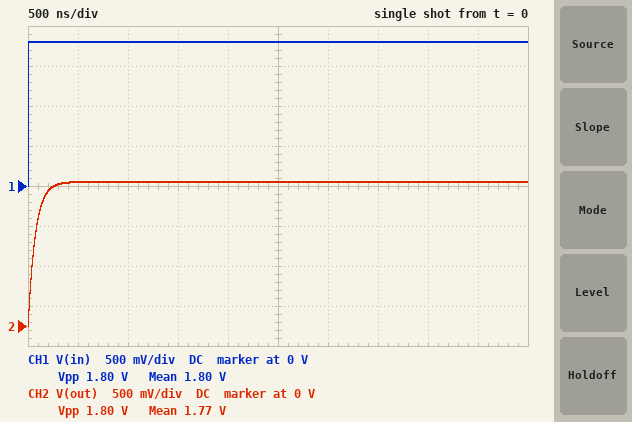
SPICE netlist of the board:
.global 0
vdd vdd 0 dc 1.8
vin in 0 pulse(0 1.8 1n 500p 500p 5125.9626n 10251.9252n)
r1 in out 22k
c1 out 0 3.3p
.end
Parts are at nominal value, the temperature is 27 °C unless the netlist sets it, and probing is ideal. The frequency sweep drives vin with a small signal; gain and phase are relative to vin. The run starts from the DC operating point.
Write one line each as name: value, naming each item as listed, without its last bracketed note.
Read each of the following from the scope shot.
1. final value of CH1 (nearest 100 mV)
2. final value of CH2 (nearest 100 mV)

final value of CH1: 1.8 V
final value of CH2: 1.8 V
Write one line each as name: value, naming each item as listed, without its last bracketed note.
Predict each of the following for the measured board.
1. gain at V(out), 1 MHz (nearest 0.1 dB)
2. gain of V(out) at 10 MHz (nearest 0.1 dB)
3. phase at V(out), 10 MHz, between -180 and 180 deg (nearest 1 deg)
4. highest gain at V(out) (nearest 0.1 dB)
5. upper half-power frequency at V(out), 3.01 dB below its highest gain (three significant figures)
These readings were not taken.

gain at V(out), 1 MHz: -0.8 dB
gain of V(out) at 10 MHz: -13.4 dB
phase at V(out), 10 MHz, between -180 and 180 deg: -78 deg
highest gain at V(out): 0 dB
upper half-power frequency at V(out), 3.01 dB below its highest gain: 2.19 MHz
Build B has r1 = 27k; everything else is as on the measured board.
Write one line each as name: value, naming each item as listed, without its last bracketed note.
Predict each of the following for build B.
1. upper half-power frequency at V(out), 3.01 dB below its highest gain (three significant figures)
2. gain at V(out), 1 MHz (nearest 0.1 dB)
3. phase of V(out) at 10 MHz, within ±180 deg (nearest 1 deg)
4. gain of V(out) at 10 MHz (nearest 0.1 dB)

upper half-power frequency at V(out), 3.01 dB below its highest gain: 1.79 MHz
gain at V(out), 1 MHz: -1.2 dB
phase of V(out) at 10 MHz, within ±180 deg: -80 deg
gain of V(out) at 10 MHz: -15.1 dB
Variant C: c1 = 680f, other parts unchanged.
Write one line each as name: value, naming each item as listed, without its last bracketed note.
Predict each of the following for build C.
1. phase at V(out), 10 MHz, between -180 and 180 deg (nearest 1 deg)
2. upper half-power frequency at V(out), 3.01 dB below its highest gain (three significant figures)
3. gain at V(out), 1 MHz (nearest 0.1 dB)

phase at V(out), 10 MHz, between -180 and 180 deg: -43 deg
upper half-power frequency at V(out), 3.01 dB below its highest gain: 10.6 MHz
gain at V(out), 1 MHz: 0 dB
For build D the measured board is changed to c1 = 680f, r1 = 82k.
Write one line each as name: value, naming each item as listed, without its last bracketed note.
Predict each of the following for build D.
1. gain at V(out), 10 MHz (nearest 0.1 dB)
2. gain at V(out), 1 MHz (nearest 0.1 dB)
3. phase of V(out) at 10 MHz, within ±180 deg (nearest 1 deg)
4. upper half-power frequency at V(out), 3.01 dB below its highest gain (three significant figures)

gain at V(out), 10 MHz: -11.2 dB
gain at V(out), 1 MHz: -0.5 dB
phase of V(out) at 10 MHz, within ±180 deg: -74 deg
upper half-power frequency at V(out), 3.01 dB below its highest gain: 2.85 MHz
